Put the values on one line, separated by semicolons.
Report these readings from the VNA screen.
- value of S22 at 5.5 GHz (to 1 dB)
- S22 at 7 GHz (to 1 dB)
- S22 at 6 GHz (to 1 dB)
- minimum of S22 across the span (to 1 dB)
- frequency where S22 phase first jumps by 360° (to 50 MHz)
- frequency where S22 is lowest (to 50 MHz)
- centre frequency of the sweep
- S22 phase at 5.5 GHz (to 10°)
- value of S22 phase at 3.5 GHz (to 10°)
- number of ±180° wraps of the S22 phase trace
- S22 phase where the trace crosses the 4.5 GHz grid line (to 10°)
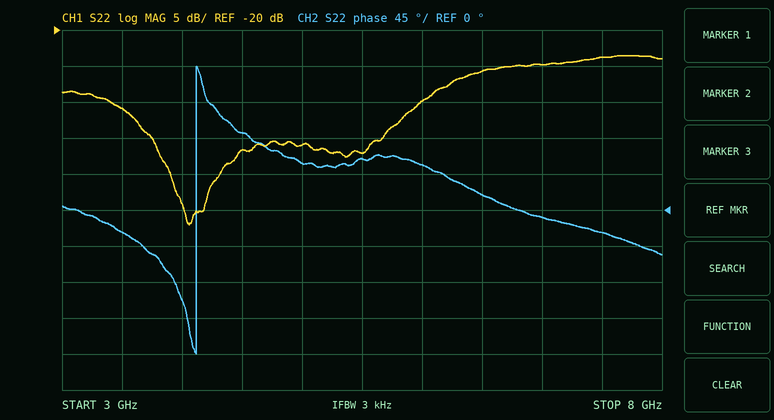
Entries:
-37 dB; -25 dB; -30 dB; -47 dB; 4.10 GHz; 4.05 GHz; 5.5 GHz; 60°; -30°; 1; 100°
